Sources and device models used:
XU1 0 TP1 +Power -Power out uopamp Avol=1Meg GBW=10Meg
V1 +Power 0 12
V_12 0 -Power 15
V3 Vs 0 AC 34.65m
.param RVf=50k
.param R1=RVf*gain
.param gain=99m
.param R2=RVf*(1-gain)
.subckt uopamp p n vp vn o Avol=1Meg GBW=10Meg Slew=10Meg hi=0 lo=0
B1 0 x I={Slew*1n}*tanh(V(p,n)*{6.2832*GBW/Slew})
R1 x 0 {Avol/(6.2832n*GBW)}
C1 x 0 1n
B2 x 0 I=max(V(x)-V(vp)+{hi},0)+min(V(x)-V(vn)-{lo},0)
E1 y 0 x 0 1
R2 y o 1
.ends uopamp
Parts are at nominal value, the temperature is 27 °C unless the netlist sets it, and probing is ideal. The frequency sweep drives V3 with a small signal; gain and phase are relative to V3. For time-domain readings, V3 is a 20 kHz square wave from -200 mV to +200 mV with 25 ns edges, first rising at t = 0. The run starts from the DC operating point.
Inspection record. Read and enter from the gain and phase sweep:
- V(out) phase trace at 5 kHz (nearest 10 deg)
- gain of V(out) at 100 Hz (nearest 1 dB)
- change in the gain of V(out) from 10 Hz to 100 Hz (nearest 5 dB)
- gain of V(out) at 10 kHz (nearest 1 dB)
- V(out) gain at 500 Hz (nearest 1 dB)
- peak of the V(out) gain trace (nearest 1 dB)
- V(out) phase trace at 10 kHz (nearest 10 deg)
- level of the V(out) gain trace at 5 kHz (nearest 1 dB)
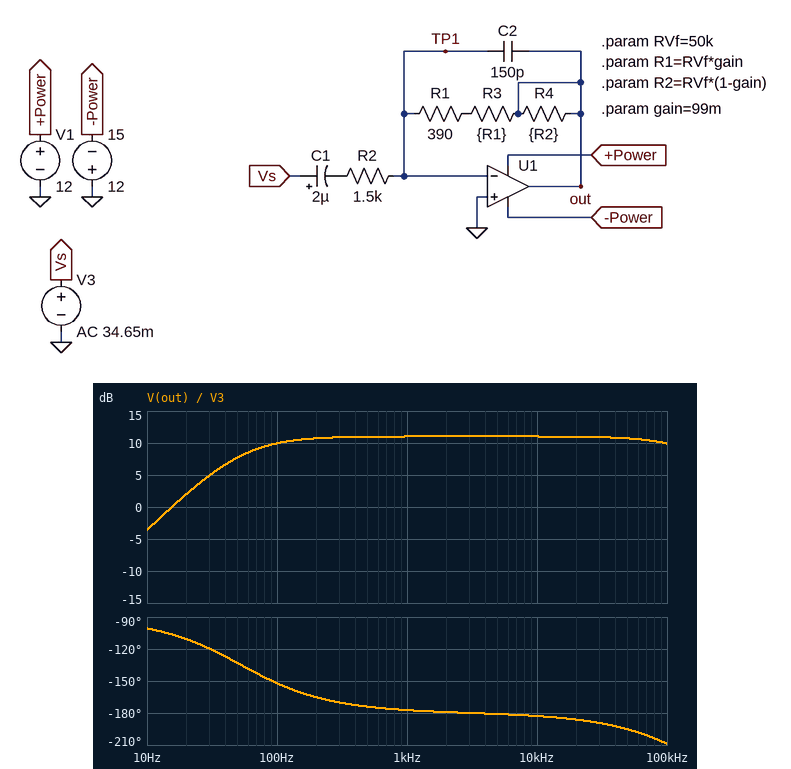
-180 deg
10 dB
15 dB
11 dB
11 dB
11 dB
-180 deg
11 dB
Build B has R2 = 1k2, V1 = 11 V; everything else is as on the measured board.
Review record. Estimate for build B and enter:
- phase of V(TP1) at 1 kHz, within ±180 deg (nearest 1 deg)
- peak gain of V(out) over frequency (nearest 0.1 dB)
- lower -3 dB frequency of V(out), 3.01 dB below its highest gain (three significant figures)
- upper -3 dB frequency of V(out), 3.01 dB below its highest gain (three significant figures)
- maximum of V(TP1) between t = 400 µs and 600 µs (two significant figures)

93 deg
13.0 dB
66.3 Hz
182 kHz
31 mV
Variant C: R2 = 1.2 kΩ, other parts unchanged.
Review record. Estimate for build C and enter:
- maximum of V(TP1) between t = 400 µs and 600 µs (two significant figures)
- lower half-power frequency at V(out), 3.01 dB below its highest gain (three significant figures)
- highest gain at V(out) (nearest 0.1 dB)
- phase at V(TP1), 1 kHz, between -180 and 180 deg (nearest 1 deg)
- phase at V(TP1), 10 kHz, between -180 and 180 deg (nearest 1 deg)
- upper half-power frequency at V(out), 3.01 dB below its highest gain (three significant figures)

31 mV
66.3 Hz
13.0 dB
93 deg
87 deg
182 kHz
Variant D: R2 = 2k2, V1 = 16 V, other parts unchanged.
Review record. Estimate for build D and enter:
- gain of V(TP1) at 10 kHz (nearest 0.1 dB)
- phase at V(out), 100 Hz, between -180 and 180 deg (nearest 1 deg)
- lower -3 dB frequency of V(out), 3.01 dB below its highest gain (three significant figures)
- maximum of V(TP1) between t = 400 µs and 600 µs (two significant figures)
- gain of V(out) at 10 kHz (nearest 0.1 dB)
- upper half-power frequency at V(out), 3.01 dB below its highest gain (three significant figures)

-52.3 dB
-160 deg
36.2 Hz
17 mV
7.7 dB
189 kHz
